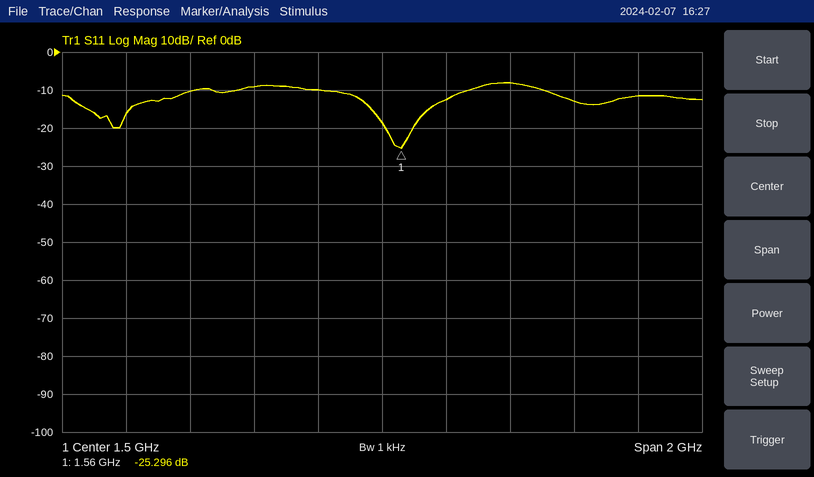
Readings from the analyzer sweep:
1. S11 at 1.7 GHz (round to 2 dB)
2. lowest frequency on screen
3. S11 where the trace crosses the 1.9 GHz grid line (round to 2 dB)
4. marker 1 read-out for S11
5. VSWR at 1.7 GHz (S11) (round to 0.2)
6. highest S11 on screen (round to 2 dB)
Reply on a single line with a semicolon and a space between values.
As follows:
-12 dB; 500 MHz; -8 dB; -25.296 dB; 1.6; -8 dB
